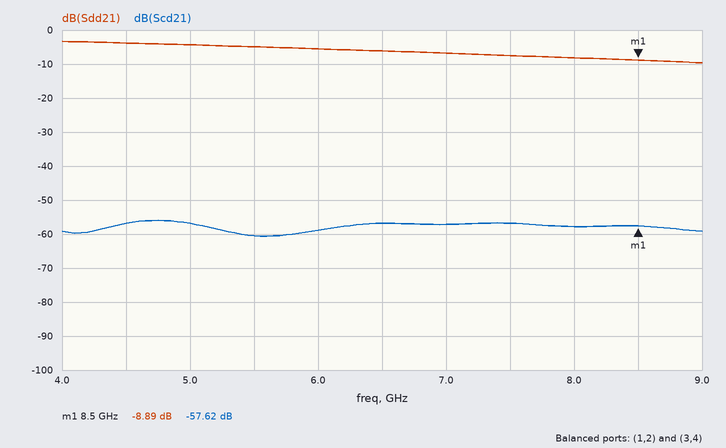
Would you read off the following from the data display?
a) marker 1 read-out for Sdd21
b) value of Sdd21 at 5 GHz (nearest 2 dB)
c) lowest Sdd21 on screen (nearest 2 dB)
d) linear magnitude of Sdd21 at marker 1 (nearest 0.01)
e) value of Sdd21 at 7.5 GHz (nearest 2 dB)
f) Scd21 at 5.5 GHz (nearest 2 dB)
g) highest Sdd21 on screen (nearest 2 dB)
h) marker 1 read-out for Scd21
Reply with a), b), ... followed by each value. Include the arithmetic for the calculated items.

a) -8.89 dB
b) -4 dB
c) -10 dB
d) 10^(-8.89/20) ≈ 0.36
e) -8 dB
f) -60 dB
g) -4 dB
h) -57.62 dB
